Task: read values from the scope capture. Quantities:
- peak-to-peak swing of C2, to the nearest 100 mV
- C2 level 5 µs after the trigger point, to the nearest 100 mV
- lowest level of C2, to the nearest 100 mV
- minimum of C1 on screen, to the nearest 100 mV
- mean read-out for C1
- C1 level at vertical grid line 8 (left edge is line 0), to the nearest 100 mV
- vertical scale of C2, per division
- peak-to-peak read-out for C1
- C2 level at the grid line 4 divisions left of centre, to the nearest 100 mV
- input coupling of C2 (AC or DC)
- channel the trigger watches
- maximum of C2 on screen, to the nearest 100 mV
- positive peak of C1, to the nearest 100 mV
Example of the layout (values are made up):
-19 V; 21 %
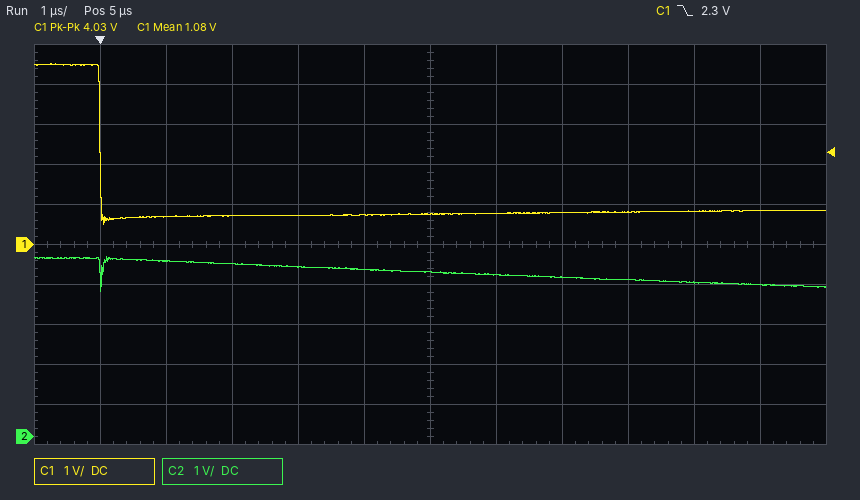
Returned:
900 mV; 4.1 V; 3.6 V; 500 mV; 1.08 V; 800 mV; 1 V; 4.03 V; 4.4 V; DC; C1; 4.5 V; 4.5 V
